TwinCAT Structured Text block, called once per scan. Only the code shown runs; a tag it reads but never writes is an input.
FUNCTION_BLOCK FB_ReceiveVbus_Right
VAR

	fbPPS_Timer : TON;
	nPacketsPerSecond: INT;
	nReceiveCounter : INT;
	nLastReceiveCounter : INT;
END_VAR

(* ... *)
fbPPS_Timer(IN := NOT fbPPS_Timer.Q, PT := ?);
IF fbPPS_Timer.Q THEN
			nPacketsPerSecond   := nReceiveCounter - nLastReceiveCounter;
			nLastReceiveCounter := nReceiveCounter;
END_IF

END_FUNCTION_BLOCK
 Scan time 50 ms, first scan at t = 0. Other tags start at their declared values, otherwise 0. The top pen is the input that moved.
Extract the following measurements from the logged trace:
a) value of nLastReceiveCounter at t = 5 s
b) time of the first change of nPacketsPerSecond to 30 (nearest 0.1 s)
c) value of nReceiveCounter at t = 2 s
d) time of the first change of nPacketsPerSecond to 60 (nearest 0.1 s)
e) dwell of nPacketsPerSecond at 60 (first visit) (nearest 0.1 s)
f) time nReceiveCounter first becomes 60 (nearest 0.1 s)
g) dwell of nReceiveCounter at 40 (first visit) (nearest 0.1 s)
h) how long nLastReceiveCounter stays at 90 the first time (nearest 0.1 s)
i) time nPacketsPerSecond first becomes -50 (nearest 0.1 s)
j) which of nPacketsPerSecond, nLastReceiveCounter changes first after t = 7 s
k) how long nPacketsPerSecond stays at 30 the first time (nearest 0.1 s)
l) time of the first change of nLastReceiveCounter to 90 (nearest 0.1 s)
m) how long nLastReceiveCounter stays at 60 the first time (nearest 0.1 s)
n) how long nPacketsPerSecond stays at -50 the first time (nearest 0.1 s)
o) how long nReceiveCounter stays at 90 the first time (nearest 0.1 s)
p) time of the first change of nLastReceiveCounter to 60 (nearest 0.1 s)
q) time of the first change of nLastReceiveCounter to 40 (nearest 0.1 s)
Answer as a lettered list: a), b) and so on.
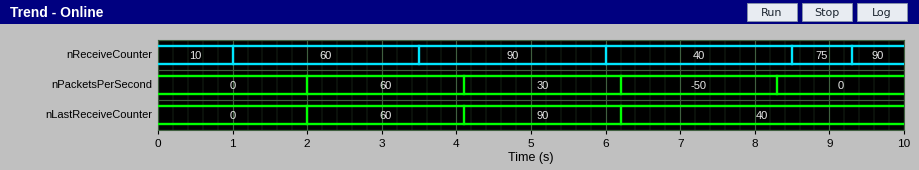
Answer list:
a) 90
b) 4.1 s
c) 60
d) 2.0 s
e) 2.1 s
f) 1.0 s
g) 2.5 s
h) 2.1 s
i) 6.2 s
j) nPacketsPerSecond
k) 2.1 s
l) 4.1 s
m) 2.1 s
n) 2.1 s
o) 2.5 s
p) 2.0 s
q) 6.2 s
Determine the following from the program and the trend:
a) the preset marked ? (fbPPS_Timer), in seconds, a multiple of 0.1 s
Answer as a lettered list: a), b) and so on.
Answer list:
a) 2.0 s
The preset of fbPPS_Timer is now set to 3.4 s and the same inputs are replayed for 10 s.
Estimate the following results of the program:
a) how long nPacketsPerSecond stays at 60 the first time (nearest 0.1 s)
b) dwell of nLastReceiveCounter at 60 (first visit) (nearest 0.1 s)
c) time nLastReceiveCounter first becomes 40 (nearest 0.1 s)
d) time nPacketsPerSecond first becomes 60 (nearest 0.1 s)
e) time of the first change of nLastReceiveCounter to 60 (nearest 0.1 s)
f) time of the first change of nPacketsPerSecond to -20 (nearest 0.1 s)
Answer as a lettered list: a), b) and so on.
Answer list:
a) 3.5 s
b) 3.5 s
c) 6.9 s
d) 3.4 s
e) 3.4 s
f) 6.9 s
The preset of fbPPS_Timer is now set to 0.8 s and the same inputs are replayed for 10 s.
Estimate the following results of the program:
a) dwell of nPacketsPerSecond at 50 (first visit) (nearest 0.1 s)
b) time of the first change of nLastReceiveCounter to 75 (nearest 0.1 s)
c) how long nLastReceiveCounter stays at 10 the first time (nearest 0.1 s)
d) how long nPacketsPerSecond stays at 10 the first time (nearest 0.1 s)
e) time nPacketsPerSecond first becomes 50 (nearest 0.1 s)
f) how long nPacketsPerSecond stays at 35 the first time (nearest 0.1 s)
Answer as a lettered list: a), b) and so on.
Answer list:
a) 0.9 s
b) 8.9 s
c) 0.9 s
d) 0.9 s
e) 1.7 s
f) 0.9 s
